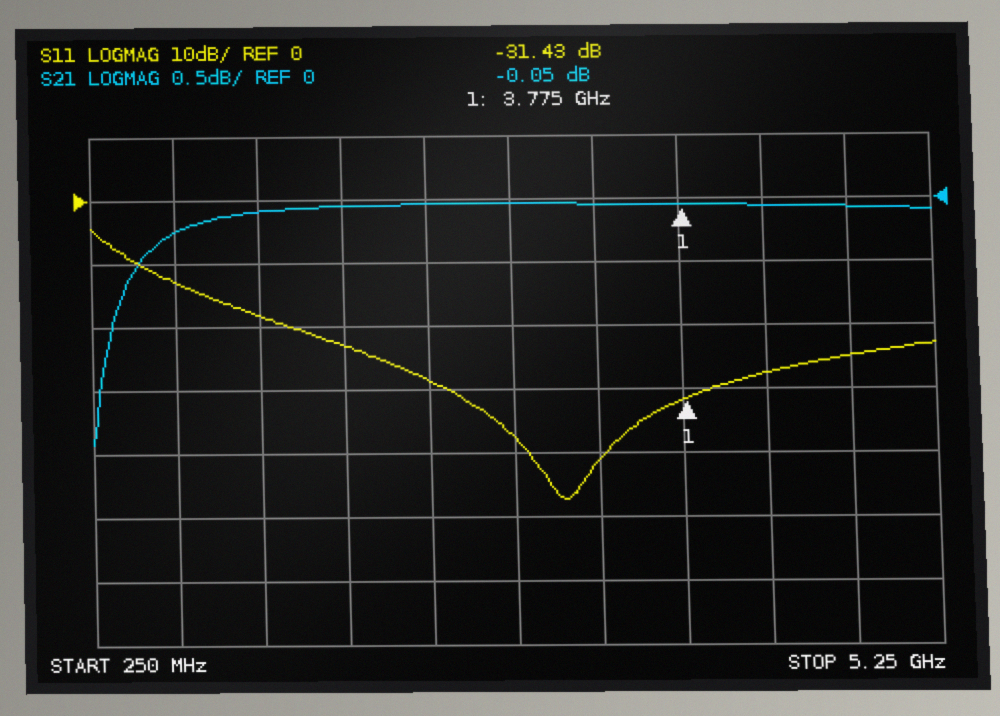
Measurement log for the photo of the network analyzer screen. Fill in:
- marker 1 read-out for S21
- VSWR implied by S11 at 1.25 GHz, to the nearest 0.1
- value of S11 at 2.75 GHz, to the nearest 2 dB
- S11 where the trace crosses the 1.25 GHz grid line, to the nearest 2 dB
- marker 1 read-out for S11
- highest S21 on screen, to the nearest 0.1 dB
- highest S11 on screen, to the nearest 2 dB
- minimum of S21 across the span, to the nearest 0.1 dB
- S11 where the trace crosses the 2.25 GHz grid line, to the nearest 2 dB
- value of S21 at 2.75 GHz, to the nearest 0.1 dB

-0.05 dB
1.3
-38 dB
-18 dB
-31.43 dB
0.0 dB
-4 dB
-1.9 dB
-28 dB
0.0 dB
